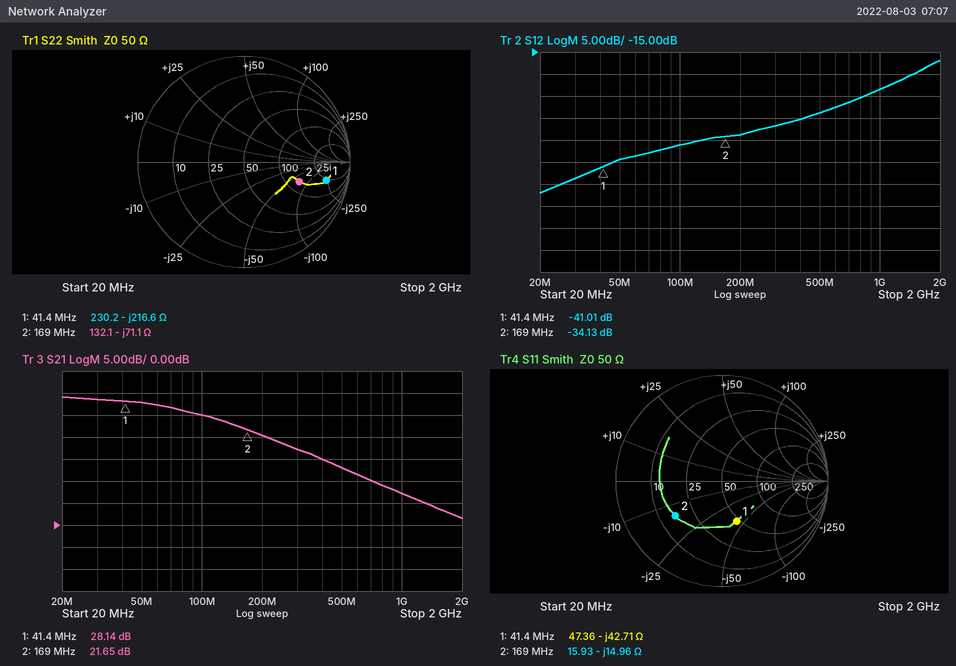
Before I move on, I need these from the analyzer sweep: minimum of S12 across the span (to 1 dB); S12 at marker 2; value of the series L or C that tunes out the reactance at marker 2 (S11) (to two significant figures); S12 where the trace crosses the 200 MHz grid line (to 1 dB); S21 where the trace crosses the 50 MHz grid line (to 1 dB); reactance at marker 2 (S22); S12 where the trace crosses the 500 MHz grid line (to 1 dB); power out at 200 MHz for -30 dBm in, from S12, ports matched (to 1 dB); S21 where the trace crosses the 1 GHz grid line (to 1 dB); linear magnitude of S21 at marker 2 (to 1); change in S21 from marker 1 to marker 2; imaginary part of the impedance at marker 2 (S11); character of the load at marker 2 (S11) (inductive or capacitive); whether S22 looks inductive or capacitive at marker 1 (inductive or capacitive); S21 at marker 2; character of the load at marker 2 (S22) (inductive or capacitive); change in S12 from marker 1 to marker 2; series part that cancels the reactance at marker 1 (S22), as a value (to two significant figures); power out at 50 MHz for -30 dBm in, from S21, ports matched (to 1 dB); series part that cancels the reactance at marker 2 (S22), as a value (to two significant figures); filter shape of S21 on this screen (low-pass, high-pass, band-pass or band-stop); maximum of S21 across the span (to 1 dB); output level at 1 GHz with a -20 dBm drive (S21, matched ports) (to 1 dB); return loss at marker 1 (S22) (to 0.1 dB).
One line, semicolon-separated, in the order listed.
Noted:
-47 dB; -34.13 dB; 14 nH; -34 dB; 28 dB; -71.1 Ω; -29 dB; -64 dBm; 7 dB; 12; -6.49 dB; -14.96 Ω; capacitive; capacitive; 21.65 dB; capacitive; 6.88 dB; 830 nH; -2 dBm; 67 nH; low-pass; 29 dB; -13 dBm; 2.0 dB
